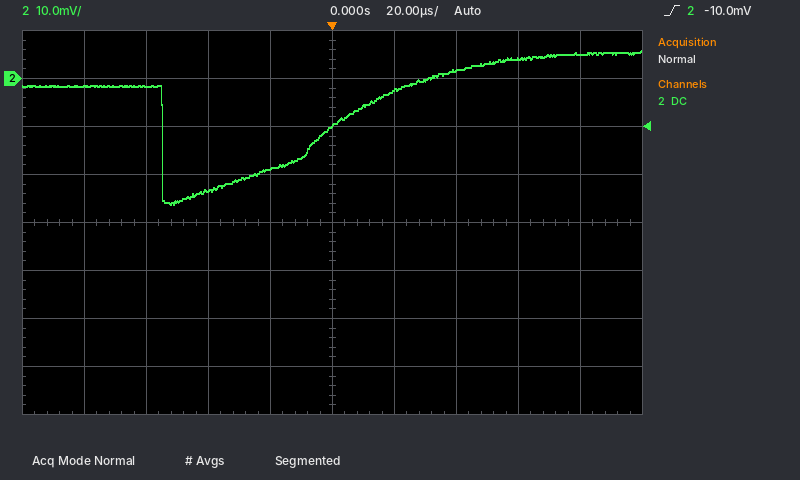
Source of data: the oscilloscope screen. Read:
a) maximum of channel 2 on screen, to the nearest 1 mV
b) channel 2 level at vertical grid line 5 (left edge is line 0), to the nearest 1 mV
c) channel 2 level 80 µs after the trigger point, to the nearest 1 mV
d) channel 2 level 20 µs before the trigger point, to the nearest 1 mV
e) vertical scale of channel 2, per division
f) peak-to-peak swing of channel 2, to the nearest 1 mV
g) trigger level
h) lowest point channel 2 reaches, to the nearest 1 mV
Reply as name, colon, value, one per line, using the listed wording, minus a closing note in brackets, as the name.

maximum of channel 2 on screen, to the nearest 1 mV: 6 mV
channel 2 level at vertical grid line 5 (left edge is line 0), to the nearest 1 mV: -10 mV
channel 2 level 80 µs after the trigger point, to the nearest 1 mV: 5 mV
channel 2 level 20 µs before the trigger point, to the nearest 1 mV: -19 mV
vertical scale of channel 2, per division: 10 mV
peak-to-peak swing of channel 2, to the nearest 1 mV: 32 mV
trigger level: -10.0 mV
lowest point channel 2 reaches, to the nearest 1 mV: -26 mV
